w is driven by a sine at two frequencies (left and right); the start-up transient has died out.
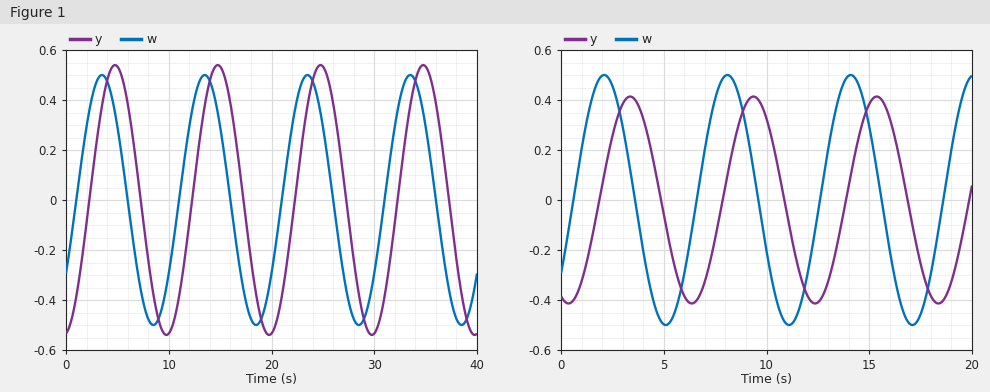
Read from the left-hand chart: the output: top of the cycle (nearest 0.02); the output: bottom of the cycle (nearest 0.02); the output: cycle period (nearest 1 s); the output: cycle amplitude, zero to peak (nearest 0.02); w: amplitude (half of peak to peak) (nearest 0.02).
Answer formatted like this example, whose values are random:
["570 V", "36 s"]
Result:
["0.54", "-0.54", "10 s", "0.54", "0.50"]
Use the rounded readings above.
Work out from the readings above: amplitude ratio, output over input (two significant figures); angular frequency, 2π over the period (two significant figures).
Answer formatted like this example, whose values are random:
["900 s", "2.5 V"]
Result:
["1.1", "0.63 rad/s"]
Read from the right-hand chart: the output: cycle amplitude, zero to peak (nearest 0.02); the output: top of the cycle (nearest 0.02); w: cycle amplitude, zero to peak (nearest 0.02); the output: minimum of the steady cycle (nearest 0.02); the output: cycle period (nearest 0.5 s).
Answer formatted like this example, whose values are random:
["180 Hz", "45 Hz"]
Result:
["0.42", "0.42", "0.50", "-0.42", "6.0 s"]
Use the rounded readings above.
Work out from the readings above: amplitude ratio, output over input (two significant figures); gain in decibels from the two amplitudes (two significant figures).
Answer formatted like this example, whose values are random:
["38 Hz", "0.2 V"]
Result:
["0.84", "-1.5 dB"]
